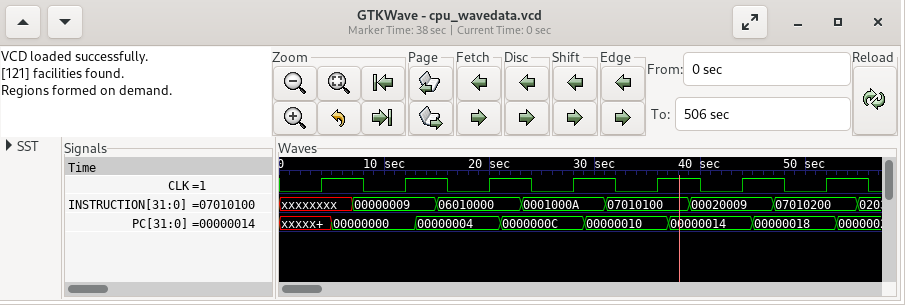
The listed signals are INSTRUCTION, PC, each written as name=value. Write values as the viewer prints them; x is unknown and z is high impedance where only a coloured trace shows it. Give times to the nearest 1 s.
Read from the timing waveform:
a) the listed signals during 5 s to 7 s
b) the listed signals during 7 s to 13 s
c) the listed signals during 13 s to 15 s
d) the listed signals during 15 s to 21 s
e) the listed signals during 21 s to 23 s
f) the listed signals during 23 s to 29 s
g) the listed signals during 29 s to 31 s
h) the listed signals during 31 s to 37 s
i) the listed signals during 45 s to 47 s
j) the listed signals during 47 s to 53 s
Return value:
INSTRUCTION=xxxxxxxx, PC=00000000
INSTRUCTION=00000009, PC=00000000
INSTRUCTION=00000009, PC=00000004
INSTRUCTION=06010000, PC=00000004
INSTRUCTION=06010000, PC=0000000C
INSTRUCTION=0001000A, PC=0000000C
INSTRUCTION=0001000A, PC=00000010
INSTRUCTION=07010100, PC=00000010
INSTRUCTION=00020009, PC=00000018
INSTRUCTION=07010200, PC=00000018
